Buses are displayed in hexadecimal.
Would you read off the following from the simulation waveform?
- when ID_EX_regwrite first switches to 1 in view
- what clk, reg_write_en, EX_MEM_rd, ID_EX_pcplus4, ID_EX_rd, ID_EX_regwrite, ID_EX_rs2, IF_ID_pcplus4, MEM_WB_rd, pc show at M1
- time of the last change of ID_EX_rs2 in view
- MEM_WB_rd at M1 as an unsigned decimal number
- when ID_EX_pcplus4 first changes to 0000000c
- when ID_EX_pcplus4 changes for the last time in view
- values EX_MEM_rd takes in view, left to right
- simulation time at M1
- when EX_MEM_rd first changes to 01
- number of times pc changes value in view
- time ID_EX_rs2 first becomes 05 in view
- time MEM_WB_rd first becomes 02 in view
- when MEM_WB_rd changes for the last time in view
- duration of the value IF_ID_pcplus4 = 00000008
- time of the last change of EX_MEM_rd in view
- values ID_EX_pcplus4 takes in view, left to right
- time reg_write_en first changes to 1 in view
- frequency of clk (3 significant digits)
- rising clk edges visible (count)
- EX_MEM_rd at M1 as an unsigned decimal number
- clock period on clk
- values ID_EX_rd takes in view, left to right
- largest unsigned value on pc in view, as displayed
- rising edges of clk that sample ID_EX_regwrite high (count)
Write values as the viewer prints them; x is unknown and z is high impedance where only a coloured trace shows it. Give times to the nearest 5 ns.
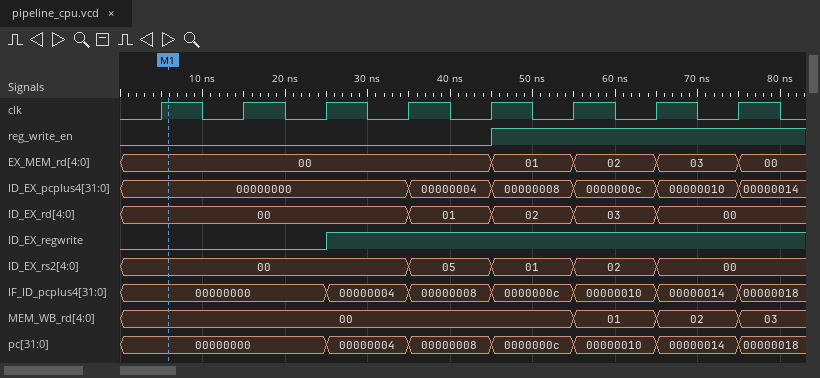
25 ns
clk=1, reg_write_en=0, EX_MEM_rd=00, ID_EX_pcplus4=00000000, ID_EX_rd=00, ID_EX_regwrite=0, ID_EX_rs2=00, IF_ID_pcplus4=00000000, MEM_WB_rd=00, pc=00000000
65 ns
0
55 ns
75 ns
00, 01, 02, 03, 00
5 ns
45 ns
6
35 ns
65 ns
75 ns
10 ns
75 ns
00000000, 00000004, 00000008, 0000000c, 00000010, 00000014
45 ns
100 MHz
8
0
10 ns
00, 01, 02, 03, 00
00000018
5
